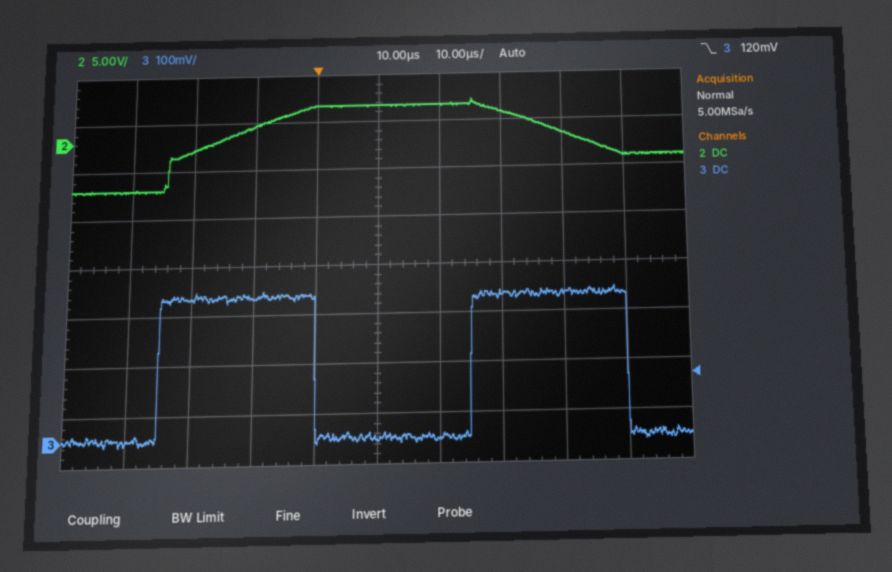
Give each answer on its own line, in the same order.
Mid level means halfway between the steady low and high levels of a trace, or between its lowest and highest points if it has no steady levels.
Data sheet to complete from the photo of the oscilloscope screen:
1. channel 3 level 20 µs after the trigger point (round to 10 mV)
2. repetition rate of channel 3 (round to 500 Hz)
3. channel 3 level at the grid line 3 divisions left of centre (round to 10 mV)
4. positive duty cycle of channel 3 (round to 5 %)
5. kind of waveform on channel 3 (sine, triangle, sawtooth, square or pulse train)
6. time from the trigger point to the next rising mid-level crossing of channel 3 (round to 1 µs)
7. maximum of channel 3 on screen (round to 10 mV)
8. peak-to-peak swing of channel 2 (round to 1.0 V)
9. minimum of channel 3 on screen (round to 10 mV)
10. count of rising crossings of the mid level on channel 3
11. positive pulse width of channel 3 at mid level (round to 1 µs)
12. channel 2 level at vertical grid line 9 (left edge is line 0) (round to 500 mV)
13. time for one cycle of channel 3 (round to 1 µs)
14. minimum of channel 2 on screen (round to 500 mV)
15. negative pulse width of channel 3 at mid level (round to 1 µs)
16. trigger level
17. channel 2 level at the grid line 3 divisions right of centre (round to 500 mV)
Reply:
0 mV
20.0 kHz
280 mV
50 %
square
25 µs
300 mV
9.0 V
-10 mV
2
25 µs
-2.0 V
50 µs
-5.0 V
25 µs
120 mV
500 mV
